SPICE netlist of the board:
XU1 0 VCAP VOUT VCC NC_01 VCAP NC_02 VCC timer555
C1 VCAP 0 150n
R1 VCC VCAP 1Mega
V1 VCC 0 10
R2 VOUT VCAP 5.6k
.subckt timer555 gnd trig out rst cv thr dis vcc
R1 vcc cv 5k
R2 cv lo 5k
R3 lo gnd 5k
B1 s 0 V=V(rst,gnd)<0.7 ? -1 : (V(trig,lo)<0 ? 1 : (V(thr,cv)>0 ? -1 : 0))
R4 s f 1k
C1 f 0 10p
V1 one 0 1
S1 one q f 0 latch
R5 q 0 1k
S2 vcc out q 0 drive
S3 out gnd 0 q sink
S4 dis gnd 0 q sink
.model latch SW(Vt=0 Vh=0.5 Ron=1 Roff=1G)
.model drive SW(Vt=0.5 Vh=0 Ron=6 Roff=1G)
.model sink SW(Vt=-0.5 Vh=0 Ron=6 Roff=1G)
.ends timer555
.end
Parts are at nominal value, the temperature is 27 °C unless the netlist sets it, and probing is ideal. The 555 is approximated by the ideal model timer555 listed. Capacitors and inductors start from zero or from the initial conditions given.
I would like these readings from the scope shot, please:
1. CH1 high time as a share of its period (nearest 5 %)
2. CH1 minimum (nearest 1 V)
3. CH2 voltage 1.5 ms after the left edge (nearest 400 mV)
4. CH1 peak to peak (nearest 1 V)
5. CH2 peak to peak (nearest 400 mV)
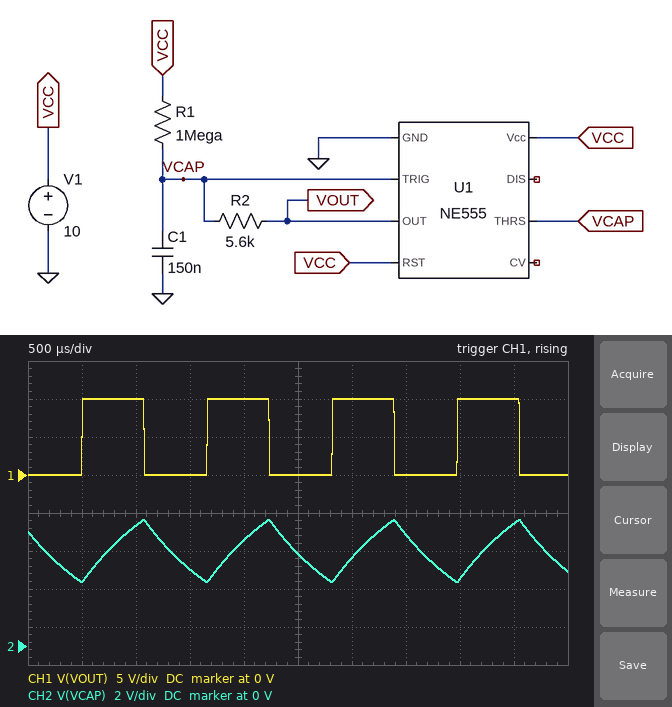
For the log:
50 %
0 V
4.0 V
10 V
3.2 V
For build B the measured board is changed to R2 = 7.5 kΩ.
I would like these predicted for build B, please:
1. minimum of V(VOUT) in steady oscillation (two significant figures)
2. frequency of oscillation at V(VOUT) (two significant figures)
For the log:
2.7 mV
640 Hz
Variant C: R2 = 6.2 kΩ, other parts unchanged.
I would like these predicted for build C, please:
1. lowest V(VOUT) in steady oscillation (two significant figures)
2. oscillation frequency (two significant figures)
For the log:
3.2 mV
770 Hz
